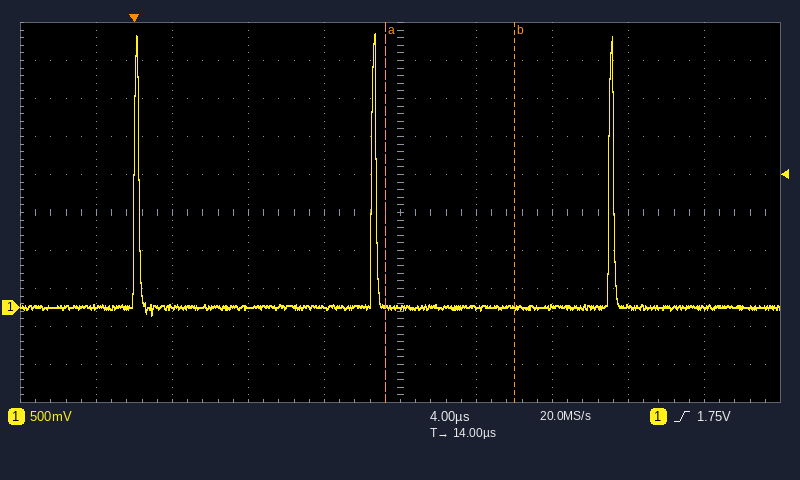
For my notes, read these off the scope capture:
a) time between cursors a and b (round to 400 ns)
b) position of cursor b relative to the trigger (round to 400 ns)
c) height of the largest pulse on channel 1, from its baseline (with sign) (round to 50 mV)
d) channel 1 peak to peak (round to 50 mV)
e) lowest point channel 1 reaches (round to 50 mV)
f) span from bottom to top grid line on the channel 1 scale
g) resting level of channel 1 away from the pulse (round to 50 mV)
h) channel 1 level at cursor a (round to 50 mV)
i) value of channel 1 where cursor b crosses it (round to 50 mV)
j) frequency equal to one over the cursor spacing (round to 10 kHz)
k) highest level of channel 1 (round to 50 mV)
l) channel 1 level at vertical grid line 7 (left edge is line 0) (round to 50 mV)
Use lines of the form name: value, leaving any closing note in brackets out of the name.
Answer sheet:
time between cursors a and b: 6.8 µs
position of cursor b relative to the trigger: +20.0 µs
height of the largest pulse on channel 1, from its baseline (with sign): +3.60 V
channel 1 peak to peak: 3.70 V
lowest point channel 1 reaches: -100 mV
span from bottom to top grid line on the channel 1 scale: 5 V
resting level of channel 1 away from the pulse: 0 mV
channel 1 level at cursor a: 0 mV
value of channel 1 where cursor b crosses it: 0 mV
frequency equal to one over the cursor spacing: 150 kHz
highest level of channel 1: 3.60 V
channel 1 level at vertical grid line 7 (left edge is line 0): 0 mV
